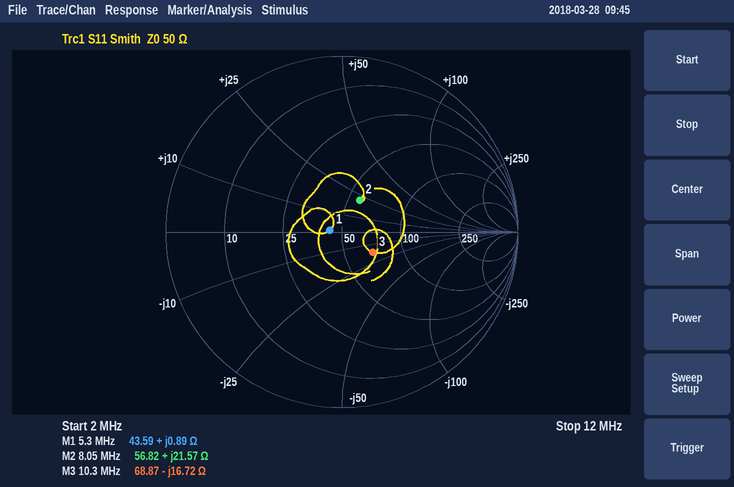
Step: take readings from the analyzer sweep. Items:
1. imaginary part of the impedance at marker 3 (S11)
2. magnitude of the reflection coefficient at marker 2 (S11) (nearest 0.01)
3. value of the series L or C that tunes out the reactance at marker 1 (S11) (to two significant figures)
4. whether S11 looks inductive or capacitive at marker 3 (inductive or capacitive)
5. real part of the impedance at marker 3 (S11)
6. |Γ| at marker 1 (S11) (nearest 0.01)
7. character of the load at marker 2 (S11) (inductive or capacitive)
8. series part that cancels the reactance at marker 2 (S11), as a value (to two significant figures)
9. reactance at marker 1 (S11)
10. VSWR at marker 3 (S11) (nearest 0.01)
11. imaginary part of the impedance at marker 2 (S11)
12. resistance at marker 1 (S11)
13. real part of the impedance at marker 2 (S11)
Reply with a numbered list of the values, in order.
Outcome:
1. -16.72 Ω
2. 0.21
3. 34 nF
4. capacitive
5. 68.87 Ω
6. 0.07
7. inductive
8. 920 pF
9. +0.89 Ω
10. 1.53
11. +21.57 Ω
12. 43.59 Ω
13. 56.82 Ω
